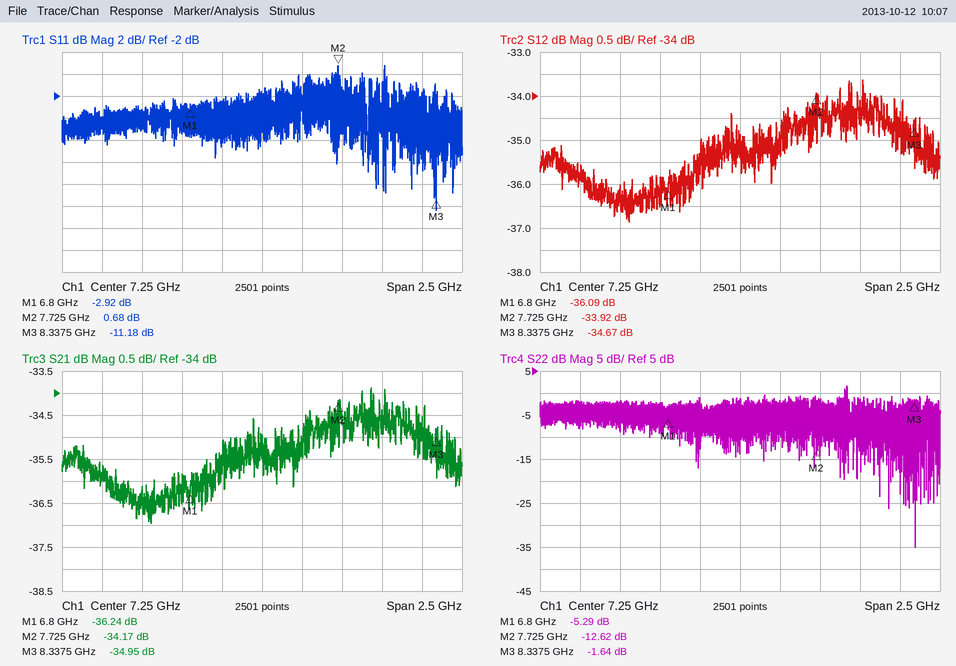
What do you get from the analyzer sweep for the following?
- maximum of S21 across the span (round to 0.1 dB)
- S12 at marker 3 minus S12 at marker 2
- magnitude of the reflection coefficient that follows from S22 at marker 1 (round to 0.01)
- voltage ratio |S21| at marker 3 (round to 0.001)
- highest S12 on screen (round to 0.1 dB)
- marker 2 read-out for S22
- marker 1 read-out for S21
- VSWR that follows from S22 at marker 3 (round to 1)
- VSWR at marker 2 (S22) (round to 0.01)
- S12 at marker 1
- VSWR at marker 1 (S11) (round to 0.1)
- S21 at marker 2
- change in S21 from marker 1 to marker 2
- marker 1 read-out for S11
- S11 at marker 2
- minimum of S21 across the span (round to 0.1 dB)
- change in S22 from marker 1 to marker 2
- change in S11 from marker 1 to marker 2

-33.9 dB
-0.75 dB
0.54
0.018
-33.6 dB
-12.62 dB
-36.24 dB
11
1.61
-36.09 dB
6.0
-34.17 dB
2.07 dB
-2.92 dB
0.68 dB
-37.0 dB
-7.33 dB
3.60 dB
